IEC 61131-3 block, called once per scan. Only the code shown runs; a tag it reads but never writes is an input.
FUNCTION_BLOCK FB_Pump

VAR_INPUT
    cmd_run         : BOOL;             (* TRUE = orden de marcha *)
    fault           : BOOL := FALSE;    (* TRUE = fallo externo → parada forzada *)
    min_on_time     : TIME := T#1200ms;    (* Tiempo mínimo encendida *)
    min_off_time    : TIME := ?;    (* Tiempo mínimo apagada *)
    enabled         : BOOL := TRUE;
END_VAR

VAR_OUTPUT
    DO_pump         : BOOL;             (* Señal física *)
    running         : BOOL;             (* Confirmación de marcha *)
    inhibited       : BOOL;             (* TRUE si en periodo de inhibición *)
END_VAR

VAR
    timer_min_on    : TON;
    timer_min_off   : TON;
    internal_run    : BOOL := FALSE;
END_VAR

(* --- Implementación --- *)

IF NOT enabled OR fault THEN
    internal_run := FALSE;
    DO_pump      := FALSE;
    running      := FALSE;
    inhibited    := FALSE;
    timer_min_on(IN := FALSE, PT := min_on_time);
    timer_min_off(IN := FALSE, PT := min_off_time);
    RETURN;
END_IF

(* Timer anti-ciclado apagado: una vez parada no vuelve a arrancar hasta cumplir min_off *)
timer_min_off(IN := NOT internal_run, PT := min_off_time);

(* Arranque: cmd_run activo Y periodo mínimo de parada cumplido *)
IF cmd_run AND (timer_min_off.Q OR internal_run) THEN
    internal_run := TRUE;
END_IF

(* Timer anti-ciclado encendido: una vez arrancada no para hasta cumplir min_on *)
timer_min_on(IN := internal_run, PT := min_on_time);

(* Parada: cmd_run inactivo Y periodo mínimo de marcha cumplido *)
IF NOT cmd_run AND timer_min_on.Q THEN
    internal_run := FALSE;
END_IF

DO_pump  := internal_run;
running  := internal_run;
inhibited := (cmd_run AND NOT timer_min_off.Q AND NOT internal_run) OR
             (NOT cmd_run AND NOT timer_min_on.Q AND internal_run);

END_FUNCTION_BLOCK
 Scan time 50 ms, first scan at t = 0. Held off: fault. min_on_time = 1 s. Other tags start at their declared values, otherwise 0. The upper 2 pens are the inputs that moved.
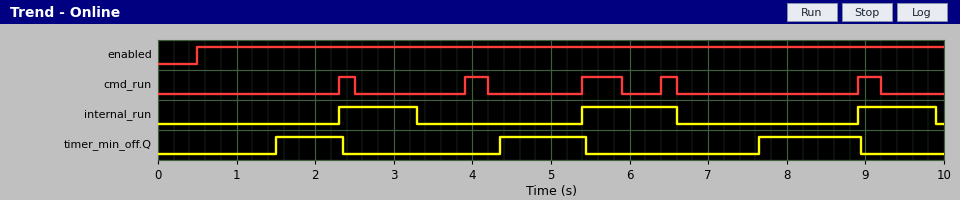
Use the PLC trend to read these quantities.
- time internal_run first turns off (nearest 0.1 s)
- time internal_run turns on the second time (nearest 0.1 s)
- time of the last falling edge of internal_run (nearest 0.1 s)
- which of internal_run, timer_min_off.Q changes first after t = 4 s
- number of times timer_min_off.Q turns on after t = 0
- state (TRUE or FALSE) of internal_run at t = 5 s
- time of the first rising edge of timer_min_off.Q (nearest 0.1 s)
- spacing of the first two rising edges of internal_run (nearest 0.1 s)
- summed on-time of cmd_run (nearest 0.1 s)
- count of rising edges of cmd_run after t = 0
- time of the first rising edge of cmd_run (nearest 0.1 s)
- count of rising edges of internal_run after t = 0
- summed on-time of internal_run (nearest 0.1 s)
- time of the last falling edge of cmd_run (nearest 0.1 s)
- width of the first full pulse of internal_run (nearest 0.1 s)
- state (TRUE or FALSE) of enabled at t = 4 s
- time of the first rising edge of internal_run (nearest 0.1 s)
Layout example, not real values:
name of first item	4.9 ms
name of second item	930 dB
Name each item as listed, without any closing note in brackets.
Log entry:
time internal_run first turns off	3.3 s
time internal_run turns on the second time	5.4 s
time of the last falling edge of internal_run	9.9 s
which of internal_run, timer_min_off.Q changes first after t = 4 s	timer_min_off.Q
number of times timer_min_off.Q turns on after t = 0	3
state (TRUE or FALSE) of internal_run at t = 5 s	FALSE
time of the first rising edge of timer_min_off.Q	1.5 s
spacing of the first two rising edges of internal_run	3.1 s
summed on-time of cmd_run	1.5 s
count of rising edges of cmd_run after t = 0	5
time of the first rising edge of cmd_run	2.3 s
count of rising edges of internal_run after t = 0	3
summed on-time of internal_run	3.2 s
time of the last falling edge of cmd_run	9.2 s
width of the first full pulse of internal_run	1.0 s
state (TRUE or FALSE) of enabled at t = 4 s	TRUE
time of the first rising edge of internal_run	2.3 s
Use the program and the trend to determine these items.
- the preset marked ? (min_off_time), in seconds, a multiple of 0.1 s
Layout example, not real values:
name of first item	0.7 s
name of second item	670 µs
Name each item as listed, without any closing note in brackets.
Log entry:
the preset marked ? (min_off_time), in seconds, a multiple of 0.1 s	1.0 s
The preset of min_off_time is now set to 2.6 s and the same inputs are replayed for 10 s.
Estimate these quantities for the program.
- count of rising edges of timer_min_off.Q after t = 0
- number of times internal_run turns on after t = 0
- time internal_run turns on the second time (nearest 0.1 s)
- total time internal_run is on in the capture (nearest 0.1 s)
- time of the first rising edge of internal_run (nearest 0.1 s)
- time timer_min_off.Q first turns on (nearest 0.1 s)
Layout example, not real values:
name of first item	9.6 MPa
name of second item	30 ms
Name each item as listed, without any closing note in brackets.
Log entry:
count of rising edges of timer_min_off.Q after t = 0	2
number of times internal_run turns on after t = 0	2
time internal_run turns on the second time	8.9 s
total time internal_run is on in the capture	2.0 s
time of the first rising edge of internal_run	3.9 s
time timer_min_off.Q first turns on	3.1 s
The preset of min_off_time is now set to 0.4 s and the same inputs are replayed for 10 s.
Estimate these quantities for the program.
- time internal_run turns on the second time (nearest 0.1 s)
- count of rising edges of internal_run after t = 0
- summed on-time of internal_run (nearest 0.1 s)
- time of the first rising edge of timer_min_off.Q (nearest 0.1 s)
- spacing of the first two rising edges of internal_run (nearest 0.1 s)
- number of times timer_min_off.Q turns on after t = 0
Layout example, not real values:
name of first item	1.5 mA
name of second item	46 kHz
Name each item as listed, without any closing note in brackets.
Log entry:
time internal_run turns on the second time	3.9 s
count of rising edges of internal_run after t = 0	4
summed on-time of internal_run	4.2 s
time of the first rising edge of timer_min_off.Q	0.9 s
spacing of the first two rising edges of internal_run	1.6 s
number of times timer_min_off.Q turns on after t = 0	4
